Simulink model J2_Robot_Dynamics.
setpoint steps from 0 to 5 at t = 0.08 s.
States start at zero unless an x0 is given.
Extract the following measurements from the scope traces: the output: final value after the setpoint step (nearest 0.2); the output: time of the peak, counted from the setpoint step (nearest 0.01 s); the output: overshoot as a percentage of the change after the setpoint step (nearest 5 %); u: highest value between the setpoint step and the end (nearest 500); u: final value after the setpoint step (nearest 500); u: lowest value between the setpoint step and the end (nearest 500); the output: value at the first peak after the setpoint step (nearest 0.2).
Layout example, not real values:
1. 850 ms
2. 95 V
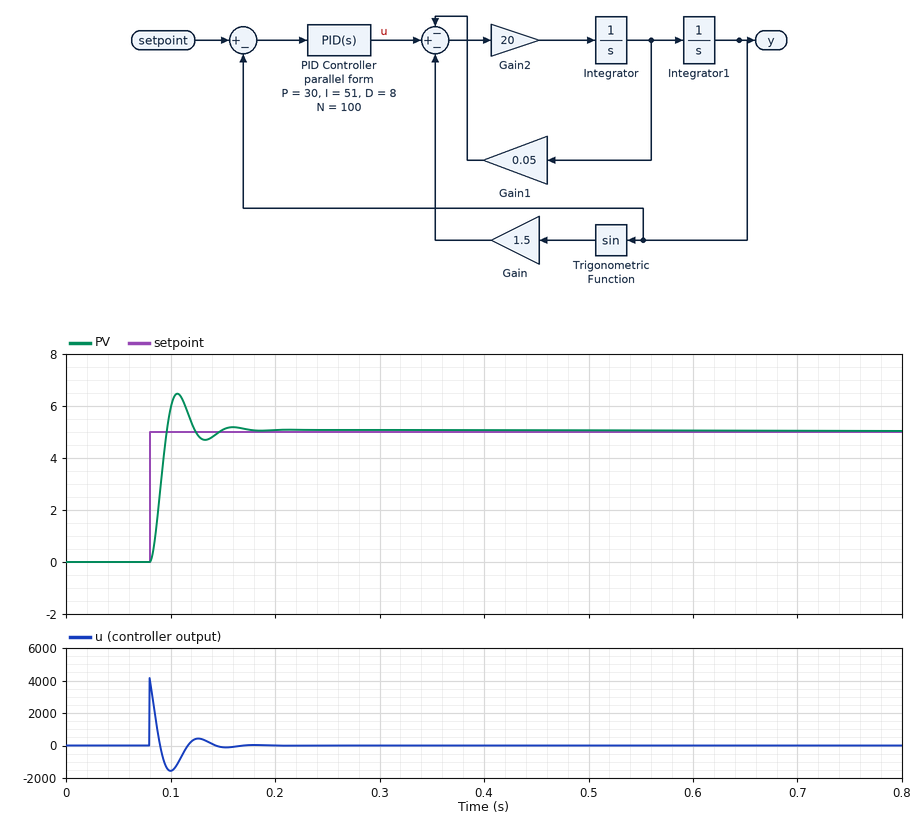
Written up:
1. 5.0
2. 0.03 s
3. 30 %
4. 4000
5. 0
6. -1500
7. 6.4
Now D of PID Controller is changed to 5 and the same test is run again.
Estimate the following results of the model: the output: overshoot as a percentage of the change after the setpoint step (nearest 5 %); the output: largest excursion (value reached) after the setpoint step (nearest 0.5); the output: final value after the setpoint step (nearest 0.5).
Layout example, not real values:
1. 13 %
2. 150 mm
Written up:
1. 25 %
2. 6.0
3. 5.0
